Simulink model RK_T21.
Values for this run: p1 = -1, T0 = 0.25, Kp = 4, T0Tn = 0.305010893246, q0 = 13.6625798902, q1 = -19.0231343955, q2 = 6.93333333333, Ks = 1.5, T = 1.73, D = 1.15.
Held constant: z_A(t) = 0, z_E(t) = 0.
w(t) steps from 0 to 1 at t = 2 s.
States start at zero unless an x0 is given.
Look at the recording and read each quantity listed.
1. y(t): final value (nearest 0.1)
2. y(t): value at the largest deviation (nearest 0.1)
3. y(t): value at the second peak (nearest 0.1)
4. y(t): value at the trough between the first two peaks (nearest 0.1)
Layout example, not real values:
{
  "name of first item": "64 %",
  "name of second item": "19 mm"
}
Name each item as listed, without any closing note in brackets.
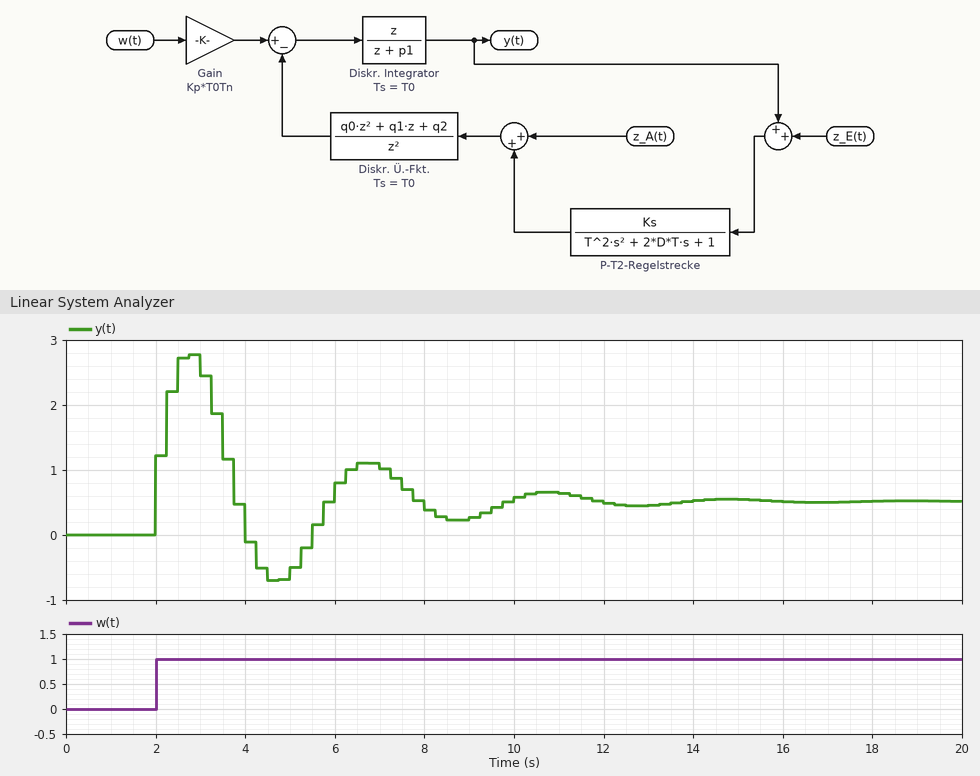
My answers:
{
  "y(t): final value": "0.5",
  "y(t): value at the largest deviation": "2.8",
  "y(t): value at the second peak": "1.1",
  "y(t): value at the trough between the first two peaks": "-0.7"
}
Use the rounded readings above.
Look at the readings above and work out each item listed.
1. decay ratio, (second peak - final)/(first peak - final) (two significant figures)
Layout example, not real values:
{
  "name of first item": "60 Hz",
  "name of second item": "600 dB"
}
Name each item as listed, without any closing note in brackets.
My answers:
{
  "decay ratio, (second peak - final)/(first peak - final)": "0.26"
}
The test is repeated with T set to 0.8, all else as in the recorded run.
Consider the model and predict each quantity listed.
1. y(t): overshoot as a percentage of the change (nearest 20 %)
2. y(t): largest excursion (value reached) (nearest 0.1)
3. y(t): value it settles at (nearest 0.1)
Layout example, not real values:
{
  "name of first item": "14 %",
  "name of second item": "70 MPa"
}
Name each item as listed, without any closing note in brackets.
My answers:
{
  "y(t): overshoot as a percentage of the change": "180 %",
  "y(t): largest excursion (value reached)": "1.5",
  "y(t): value it settles at": "0.5"
}
